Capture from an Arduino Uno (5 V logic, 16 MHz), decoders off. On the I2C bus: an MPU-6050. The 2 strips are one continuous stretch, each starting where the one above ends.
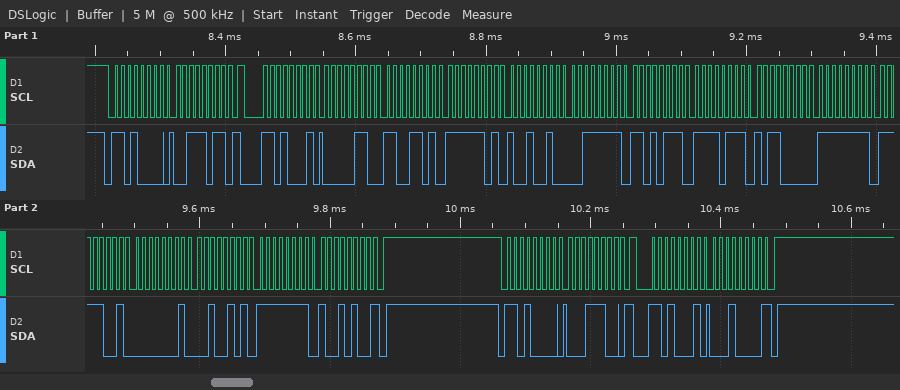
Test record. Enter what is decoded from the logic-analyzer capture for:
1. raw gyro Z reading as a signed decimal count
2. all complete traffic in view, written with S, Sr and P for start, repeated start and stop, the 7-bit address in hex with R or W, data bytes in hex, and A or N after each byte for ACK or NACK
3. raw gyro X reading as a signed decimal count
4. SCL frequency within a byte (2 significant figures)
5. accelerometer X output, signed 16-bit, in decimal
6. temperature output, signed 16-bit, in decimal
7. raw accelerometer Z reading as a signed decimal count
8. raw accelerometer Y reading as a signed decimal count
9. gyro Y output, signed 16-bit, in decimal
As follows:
-108
S 68W A 3B A Sr 68R A 06 A CD A FD A 92 A 3F A D7 A F7 A B0 A FF A F9 A 01 A 25 A FF A 94 N P S 68W A 1C A Sr 68R A 10 N P
-7
100 kHz
1741
-2128
16343
-622
293
